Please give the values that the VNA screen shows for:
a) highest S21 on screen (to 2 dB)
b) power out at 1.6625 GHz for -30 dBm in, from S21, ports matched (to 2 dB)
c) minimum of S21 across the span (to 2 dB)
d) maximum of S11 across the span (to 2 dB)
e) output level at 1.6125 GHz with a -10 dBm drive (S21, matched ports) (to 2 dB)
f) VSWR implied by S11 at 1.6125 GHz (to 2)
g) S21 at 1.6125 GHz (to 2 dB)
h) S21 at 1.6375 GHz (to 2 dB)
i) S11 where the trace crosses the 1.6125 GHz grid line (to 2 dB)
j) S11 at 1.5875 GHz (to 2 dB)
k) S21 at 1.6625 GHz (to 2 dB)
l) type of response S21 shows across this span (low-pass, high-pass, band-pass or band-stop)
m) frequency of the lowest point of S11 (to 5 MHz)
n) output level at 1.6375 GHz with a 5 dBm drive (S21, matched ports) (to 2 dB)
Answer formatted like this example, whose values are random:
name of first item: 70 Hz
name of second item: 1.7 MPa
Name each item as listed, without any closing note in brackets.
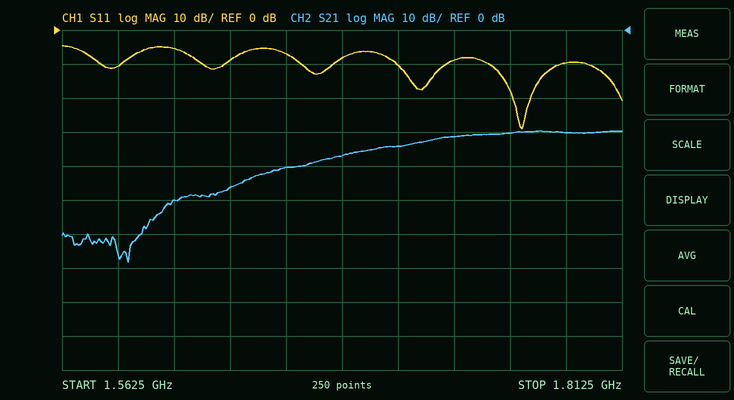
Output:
highest S21 on screen: -30 dB
power out at 1.6625 GHz for -30 dBm in, from S21, ports matched: -70 dBm
minimum of S21 across the span: -68 dB
maximum of S11 across the span: -4 dB
output level at 1.6125 GHz with a -10 dBm drive (S21, matched ports): -60 dBm
VSWR implied by S11 at 1.6125 GHz: 4
S21 at 1.6125 GHz: -50 dB
S21 at 1.6375 GHz: -46 dB
S11 where the trace crosses the 1.6125 GHz grid line: -6 dB
S11 at 1.5875 GHz: -10 dB
S21 at 1.6625 GHz: -40 dB
type of response S21 shows across this span: high-pass
frequency of the lowest point of S11: 1.770 GHz
output level at 1.6375 GHz with a 5 dBm drive (S21, matched ports): -42 dBm
